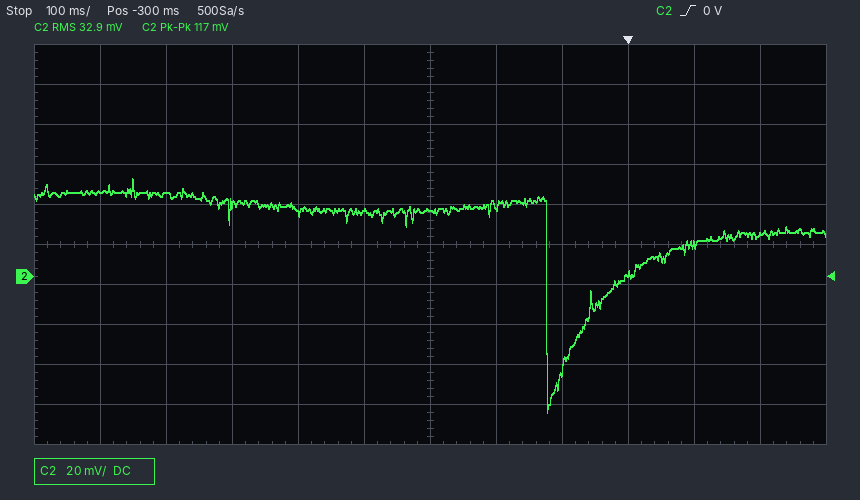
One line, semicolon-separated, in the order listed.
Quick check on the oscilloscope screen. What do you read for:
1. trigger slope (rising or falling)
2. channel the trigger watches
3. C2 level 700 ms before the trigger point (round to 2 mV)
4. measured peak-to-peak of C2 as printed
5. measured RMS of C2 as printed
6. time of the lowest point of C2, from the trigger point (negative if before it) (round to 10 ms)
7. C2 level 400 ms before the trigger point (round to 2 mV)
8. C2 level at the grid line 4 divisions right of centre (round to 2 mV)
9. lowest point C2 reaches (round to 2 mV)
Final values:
rising; C2; 42 mV; 117 mV; 32.9 mV; -120 ms; 32 mV; 16 mV; -68 mV
